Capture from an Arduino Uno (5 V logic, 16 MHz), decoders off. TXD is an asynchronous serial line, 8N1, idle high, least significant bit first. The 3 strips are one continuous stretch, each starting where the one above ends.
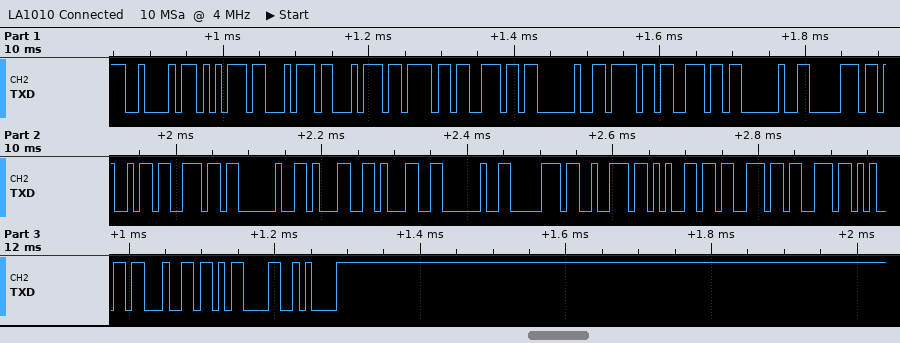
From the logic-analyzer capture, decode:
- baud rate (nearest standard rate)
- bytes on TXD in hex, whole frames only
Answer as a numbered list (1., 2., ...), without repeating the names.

1. 115200 baud
2. 42 75 74 74 6F 6E 20 6F 6E 20 70 69 6E 20 31 31 20 70 72 65 73 73 65 64 0D 0A
